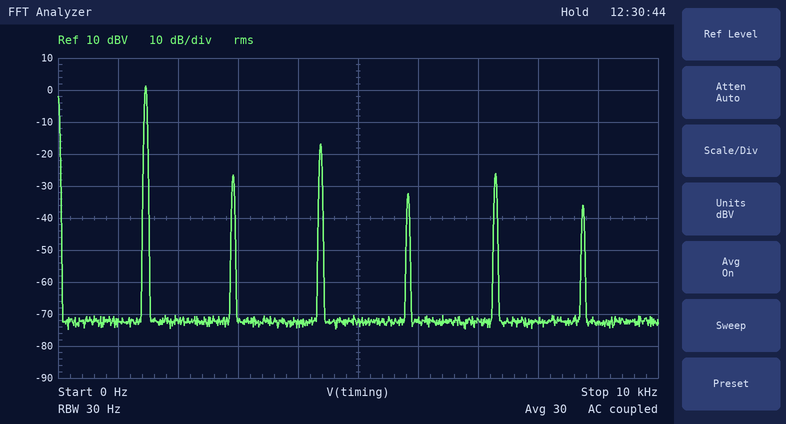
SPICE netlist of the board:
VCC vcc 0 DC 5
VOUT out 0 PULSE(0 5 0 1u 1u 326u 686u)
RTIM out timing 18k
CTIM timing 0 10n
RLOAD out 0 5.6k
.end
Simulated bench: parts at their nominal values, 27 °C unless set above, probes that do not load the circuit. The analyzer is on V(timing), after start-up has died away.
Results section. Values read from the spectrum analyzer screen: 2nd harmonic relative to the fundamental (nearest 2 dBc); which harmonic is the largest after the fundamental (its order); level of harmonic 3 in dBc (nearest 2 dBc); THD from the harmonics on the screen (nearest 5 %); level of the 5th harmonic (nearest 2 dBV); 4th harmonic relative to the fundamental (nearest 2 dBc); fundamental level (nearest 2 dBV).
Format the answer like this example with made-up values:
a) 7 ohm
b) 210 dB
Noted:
a) -28 dBc
b) 3
c) -18 dBc
d) 15 %
e) -26 dBV
f) -34 dBc
g) 2 dBV
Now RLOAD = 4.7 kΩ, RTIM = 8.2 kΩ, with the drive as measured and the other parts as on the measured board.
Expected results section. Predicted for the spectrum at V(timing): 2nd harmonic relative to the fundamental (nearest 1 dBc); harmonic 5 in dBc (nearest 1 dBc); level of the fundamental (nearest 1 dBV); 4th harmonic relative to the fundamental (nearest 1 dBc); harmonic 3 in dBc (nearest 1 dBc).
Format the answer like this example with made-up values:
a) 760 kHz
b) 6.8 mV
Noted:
a) -26 dBc
b) -24 dBc
c) 5 dBV
d) -31 dBc
e) -16 dBc
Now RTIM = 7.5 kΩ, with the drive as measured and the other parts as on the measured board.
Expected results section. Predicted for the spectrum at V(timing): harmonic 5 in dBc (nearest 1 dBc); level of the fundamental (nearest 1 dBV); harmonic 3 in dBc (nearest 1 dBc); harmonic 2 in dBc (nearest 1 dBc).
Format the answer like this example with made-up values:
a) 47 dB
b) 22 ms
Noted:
a) -24 dBc
b) 5 dBV
c) -15 dBc
d) -26 dBc
